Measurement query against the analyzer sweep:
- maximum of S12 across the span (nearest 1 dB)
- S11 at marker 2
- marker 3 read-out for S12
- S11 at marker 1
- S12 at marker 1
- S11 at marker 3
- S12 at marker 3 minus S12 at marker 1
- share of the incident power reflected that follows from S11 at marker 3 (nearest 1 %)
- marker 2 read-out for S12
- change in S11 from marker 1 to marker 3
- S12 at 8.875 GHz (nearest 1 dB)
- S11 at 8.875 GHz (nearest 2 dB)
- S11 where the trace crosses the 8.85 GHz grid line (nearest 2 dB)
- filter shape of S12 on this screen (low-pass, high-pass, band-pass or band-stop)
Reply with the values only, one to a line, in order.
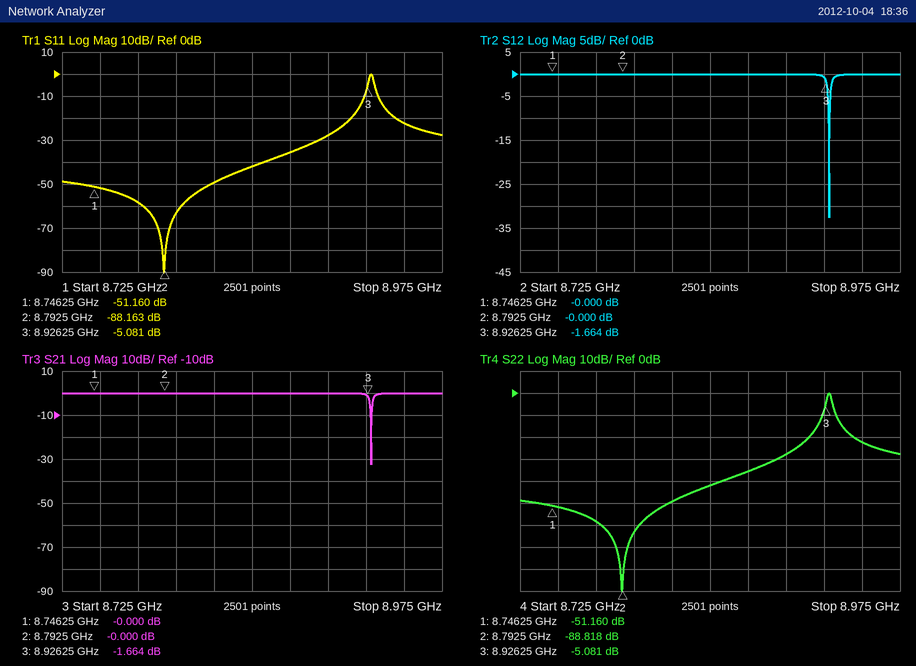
0 dB
-88.163 dB
-1.664 dB
-51.160 dB
-0.000 dB
-5.081 dB
-1.664 dB
31 %
-0.000 dB
46.079 dB
0 dB
-36 dB
-42 dB
band-stop
